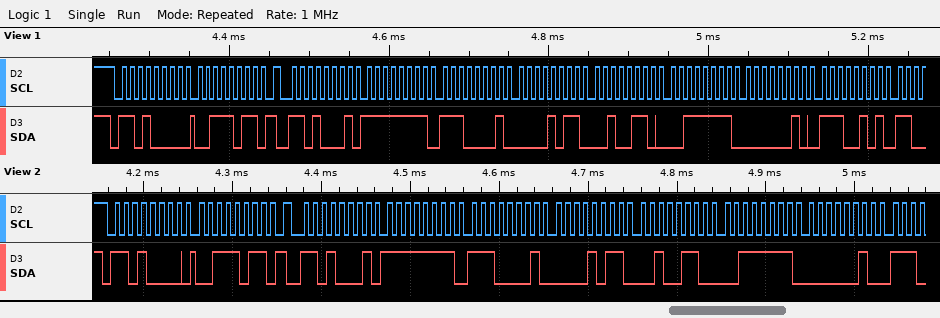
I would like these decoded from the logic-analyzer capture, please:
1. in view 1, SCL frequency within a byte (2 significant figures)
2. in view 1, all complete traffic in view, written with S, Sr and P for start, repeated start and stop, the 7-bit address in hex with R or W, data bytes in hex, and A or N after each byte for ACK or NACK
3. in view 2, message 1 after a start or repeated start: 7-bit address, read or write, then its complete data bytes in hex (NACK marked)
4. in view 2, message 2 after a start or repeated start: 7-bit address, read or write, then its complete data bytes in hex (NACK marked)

100 kHz
S 68W A 3B A Sr 68R A FF A E1 A 0B A 26 A 3F A 02 A E5 A
0x68 write: 3B
0x68 read: FF E1 0B 26 3F 02
